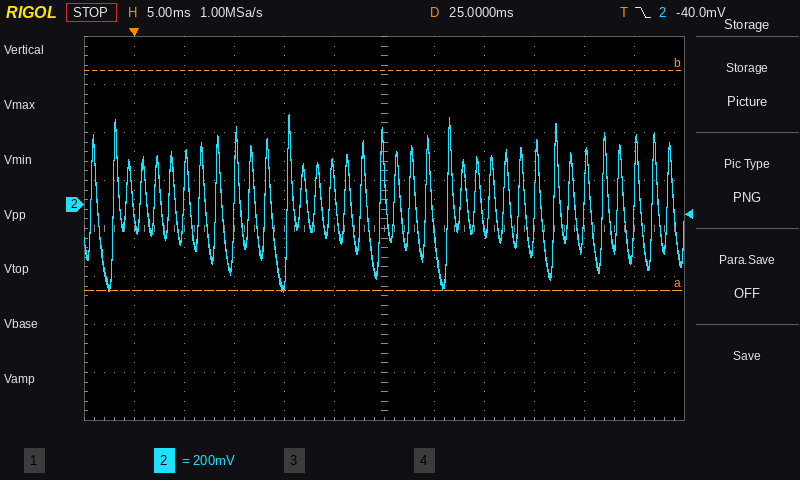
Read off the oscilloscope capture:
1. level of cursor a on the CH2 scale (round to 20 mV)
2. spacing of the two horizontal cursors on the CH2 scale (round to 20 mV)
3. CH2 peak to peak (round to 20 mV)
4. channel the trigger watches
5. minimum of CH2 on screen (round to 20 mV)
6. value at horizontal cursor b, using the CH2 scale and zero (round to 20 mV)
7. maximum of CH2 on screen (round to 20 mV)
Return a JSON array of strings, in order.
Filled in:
["-360 mV", "920 mV", "740 mV", "CH2", "-360 mV", "560 mV", "380 mV"]
